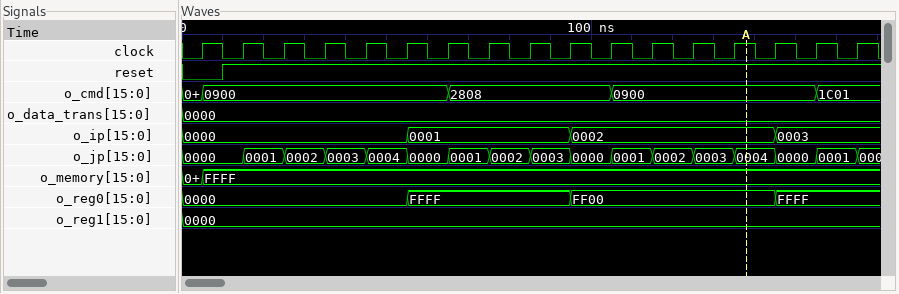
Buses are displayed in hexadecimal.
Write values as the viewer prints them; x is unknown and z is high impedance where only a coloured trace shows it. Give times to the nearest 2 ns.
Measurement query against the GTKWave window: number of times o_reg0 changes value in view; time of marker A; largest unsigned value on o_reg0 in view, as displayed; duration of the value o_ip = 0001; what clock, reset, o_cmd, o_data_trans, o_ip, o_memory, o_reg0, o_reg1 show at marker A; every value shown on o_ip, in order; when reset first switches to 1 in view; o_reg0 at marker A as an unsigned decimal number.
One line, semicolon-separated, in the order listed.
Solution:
3; 138 ns; FFFF; 40 ns; clock=1, reset=1, o_cmd=0900, o_data_trans=0000, o_ip=0002, o_memory=FFFF, o_reg0=FF00, o_reg1=0000; 0000, 0001, 0002, 0003; 10 ns; 65280
